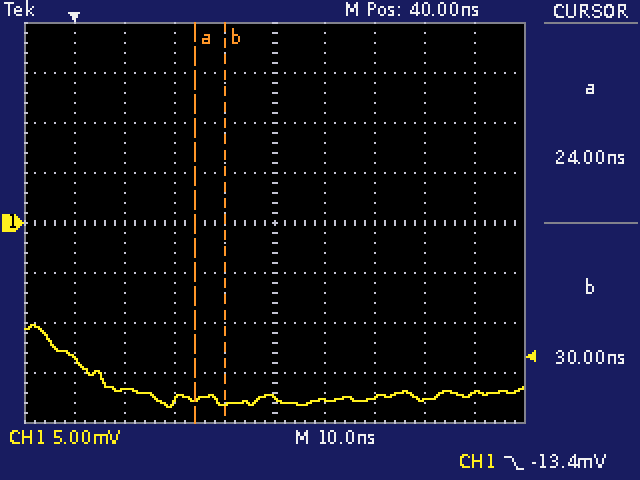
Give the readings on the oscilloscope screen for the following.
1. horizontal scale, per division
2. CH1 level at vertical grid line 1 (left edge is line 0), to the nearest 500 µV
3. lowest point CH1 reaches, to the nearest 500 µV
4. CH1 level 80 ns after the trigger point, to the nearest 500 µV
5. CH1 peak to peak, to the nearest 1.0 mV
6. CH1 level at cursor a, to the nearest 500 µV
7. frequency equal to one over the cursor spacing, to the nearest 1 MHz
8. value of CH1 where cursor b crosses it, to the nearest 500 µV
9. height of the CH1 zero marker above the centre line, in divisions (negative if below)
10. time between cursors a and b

10 ns
-13.5 mV
-18.5 mV
-17.0 mV
8.0 mV
-17.5 mV
167 MHz
-18.0 mV
0.0 div
6 ns
